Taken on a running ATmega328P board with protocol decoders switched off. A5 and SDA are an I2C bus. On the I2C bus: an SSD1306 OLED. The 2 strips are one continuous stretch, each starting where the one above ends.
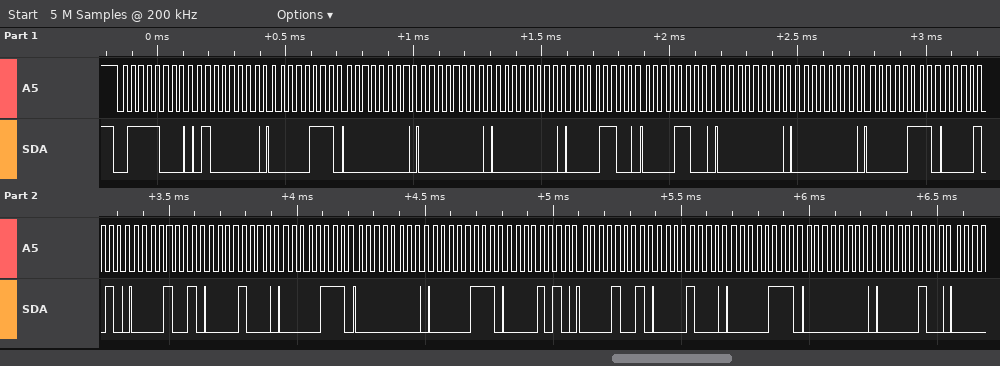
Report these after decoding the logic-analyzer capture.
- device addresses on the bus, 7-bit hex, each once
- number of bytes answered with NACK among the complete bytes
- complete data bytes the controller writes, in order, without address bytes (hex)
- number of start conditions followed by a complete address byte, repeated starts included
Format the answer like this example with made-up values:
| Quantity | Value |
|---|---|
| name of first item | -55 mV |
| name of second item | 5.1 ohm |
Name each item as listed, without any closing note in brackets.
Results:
| Quantity | Value |
|---|---|
| device addresses on the bus, 7-bit hex, each once | 0x3C |
| number of bytes answered with NACK among the complete bytes | 0 |
| complete data bytes the controller writes, in order, without address bytes | 40 07 00 00 00 0C 0C 00 00 07 0A 09 08 07 00 07 0A 09 08 07 00 04 |
| number of start conditions followed by a complete address byte, repeated starts included | 1 |
